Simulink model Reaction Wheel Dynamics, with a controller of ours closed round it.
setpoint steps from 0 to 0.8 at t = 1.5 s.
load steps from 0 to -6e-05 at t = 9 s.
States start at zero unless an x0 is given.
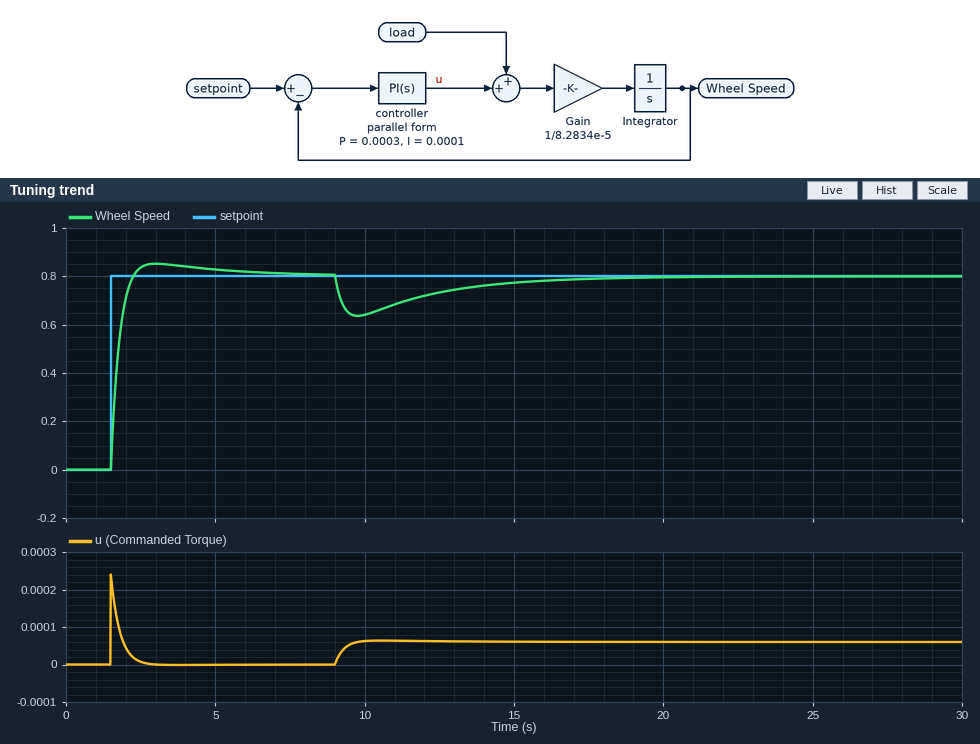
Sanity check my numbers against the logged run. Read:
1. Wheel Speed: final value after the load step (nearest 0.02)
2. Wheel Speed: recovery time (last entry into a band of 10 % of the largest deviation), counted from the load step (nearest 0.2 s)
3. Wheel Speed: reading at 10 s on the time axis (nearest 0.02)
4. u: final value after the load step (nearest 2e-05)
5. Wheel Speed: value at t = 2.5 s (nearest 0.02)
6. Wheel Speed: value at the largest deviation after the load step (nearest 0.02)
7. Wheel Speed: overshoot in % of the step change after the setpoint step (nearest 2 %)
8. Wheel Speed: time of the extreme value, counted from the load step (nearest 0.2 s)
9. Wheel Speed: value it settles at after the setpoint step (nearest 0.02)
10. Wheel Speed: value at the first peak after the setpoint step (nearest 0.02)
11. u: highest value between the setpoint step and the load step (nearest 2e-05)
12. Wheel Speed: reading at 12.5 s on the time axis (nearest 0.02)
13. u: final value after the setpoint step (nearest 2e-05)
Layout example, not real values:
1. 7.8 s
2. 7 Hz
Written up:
1. 0.80
2. 7.2 s
3. 0.64
4. 0.00006
5. 0.84
6. 0.64
7. 6 %
8. 0.8 s
9. 0.80
10. 0.86
11. 0.00024
12. 0.74
13. 0.00000
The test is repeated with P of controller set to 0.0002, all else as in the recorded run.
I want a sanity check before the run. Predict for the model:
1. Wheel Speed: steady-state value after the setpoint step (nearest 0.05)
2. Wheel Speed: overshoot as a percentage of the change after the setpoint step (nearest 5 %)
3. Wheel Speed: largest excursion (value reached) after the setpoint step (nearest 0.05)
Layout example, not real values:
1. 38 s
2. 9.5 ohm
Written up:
1. 0.80
2. 10 %
3. 0.90
